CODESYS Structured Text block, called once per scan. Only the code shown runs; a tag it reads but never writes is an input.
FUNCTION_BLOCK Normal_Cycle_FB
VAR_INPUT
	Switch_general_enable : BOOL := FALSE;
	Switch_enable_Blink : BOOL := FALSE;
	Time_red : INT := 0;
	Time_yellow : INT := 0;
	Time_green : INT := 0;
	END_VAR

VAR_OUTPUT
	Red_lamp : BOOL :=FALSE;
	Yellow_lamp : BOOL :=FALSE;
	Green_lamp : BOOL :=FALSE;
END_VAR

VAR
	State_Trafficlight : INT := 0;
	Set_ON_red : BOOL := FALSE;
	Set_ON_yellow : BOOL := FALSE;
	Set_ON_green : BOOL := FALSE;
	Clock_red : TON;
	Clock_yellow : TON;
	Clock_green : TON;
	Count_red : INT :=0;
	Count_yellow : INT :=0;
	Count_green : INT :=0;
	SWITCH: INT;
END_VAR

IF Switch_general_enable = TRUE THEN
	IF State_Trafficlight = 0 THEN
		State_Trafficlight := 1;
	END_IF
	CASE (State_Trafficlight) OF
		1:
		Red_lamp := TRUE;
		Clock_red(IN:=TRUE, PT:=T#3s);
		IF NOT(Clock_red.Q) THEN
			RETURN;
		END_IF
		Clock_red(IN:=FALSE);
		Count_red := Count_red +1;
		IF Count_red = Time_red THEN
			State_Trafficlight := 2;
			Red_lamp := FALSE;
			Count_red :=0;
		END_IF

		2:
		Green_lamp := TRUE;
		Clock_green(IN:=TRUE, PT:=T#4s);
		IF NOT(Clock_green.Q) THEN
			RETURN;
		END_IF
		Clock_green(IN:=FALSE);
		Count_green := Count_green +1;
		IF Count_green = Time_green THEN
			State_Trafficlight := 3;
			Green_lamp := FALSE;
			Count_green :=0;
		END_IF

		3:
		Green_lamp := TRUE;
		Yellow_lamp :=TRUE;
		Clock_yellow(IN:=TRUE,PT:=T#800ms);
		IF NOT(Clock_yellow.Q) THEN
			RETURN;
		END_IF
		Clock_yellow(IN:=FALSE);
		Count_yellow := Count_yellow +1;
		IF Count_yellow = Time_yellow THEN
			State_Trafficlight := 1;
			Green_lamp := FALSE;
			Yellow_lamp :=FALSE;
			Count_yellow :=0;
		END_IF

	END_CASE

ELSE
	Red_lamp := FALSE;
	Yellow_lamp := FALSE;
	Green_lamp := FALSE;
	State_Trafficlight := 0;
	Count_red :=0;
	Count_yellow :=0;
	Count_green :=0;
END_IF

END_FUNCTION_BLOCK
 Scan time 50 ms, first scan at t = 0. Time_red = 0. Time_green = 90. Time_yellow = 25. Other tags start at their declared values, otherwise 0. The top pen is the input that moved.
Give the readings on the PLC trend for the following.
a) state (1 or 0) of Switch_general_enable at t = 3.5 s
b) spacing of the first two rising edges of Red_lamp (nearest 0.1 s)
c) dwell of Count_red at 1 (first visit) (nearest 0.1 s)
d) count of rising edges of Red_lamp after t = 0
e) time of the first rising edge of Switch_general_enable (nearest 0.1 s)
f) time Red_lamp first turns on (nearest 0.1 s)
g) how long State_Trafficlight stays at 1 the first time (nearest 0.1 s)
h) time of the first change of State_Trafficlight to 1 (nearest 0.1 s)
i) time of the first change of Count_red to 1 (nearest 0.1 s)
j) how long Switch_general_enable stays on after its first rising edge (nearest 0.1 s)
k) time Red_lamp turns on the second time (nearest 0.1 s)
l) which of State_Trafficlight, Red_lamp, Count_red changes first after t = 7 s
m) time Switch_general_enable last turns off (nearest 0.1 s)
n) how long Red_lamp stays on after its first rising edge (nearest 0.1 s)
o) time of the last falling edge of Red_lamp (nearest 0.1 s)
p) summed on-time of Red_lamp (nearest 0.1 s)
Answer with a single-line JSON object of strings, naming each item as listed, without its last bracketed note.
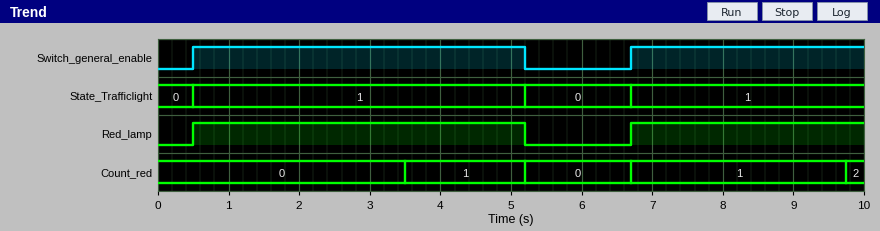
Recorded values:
{"state (1 or 0) of Switch_general_enable at t = 3.5 s": "1", "spacing of the first two rising edges of Red_lamp": "6.2 s", "dwell of Count_red at 1 (first visit)": "1.7 s", "count of rising edges of Red_lamp after t = 0": "2", "time of the first rising edge of Switch_general_enable": "0.5 s", "time Red_lamp first turns on": "0.5 s", "how long State_Trafficlight stays at 1 the first time": "4.7 s", "time of the first change of State_Trafficlight to 1": "0.5 s", "time of the first change of Count_red to 1": "3.5 s", "how long Switch_general_enable stays on after its first rising edge": "4.7 s", "time Red_lamp turns on the second time": "6.7 s", "which of State_Trafficlight, Red_lamp, Count_red changes first after t = 7 s": "Count_red", "time Switch_general_enable last turns off": "5.2 s", "how long Red_lamp stays on after its first rising edge": "4.7 s", "time of the last falling edge of Red_lamp": "5.2 s", "summed on-time of Red_lamp": "8.0 s"}
